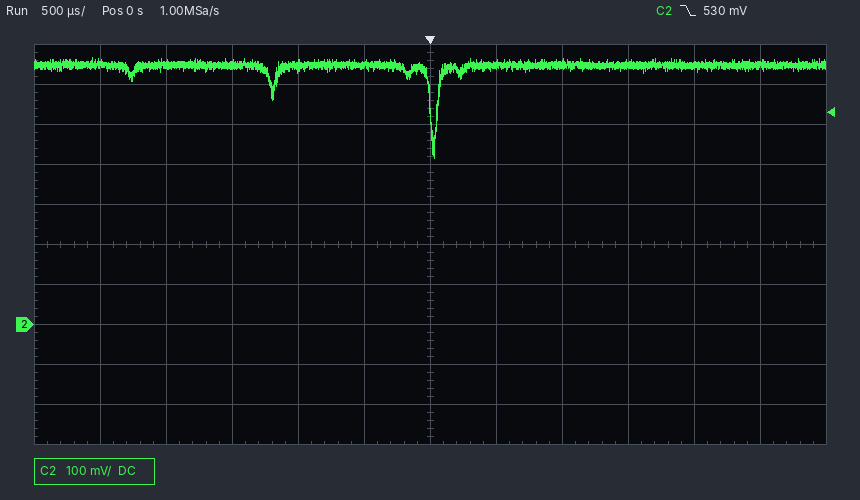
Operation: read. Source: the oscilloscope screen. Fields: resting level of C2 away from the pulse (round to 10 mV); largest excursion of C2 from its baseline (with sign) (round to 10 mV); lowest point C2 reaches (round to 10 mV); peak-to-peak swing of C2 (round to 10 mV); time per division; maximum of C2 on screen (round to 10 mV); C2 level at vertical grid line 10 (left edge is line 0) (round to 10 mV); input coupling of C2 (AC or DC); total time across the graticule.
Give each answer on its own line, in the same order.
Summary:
650 mV
-230 mV
420 mV
250 mV
500 µs
670 mV
650 mV
DC
6 ms
